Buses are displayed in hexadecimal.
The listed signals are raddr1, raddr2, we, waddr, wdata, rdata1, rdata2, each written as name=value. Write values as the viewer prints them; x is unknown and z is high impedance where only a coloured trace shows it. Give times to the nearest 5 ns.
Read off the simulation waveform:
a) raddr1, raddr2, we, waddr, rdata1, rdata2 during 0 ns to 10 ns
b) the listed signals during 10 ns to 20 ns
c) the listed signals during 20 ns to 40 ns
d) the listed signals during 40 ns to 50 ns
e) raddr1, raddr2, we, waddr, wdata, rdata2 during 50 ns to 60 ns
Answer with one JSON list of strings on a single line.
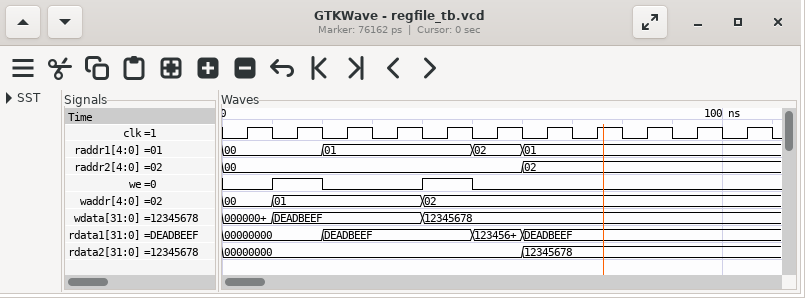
["raddr1=00, raddr2=00, we=0, waddr=00, rdata1=00000000, rdata2=00000000", "raddr1=00, raddr2=00, we=1, waddr=01, wdata=DEADBEEF, rdata1=00000000, rdata2=00000000", "raddr1=01, raddr2=00, we=0, waddr=01, wdata=DEADBEEF, rdata1=DEADBEEF, rdata2=00000000", "raddr1=01, raddr2=00, we=1, waddr=02, wdata=12345678, rdata1=DEADBEEF, rdata2=00000000", "raddr1=02, raddr2=00, we=0, waddr=02, wdata=12345678, rdata2=00000000"]
